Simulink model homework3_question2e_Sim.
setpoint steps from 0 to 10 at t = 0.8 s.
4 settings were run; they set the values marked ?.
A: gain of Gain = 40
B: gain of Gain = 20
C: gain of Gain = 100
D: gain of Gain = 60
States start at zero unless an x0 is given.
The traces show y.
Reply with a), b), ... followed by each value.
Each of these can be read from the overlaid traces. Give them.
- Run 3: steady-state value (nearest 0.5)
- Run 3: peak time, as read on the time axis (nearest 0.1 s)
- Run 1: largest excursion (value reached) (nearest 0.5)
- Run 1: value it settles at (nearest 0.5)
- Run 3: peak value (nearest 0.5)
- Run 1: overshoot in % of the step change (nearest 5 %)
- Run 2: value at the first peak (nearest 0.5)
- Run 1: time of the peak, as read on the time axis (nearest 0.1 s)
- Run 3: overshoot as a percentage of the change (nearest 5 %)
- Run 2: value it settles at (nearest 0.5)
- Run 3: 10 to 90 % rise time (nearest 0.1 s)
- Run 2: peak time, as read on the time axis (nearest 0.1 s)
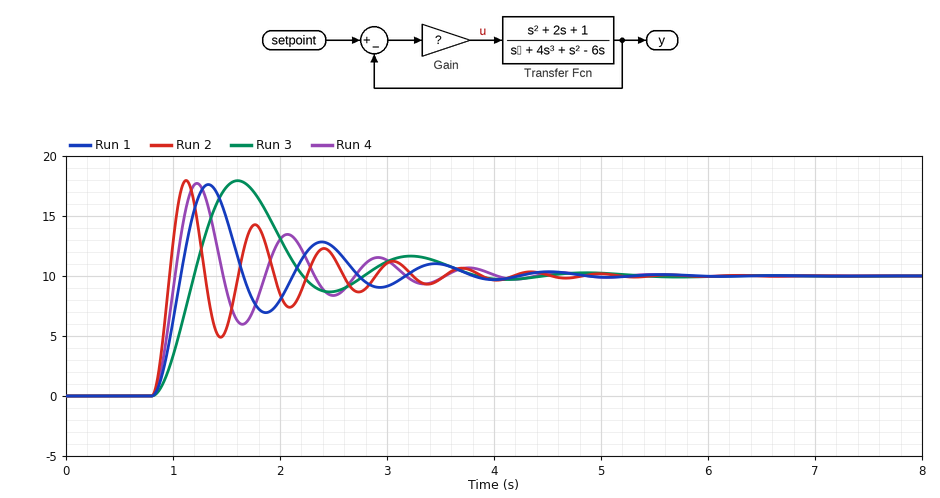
a) 10.0
b) 1.6 s
c) 17.5
d) 10.0
e) 18.0
f) 75 %
g) 18.0
h) 1.3 s
i) 80 %
j) 10.0
k) 0.3 s
l) 1.1 s
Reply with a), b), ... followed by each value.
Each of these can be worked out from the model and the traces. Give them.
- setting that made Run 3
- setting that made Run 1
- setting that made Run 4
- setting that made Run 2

a) B
b) A
c) D
d) C
